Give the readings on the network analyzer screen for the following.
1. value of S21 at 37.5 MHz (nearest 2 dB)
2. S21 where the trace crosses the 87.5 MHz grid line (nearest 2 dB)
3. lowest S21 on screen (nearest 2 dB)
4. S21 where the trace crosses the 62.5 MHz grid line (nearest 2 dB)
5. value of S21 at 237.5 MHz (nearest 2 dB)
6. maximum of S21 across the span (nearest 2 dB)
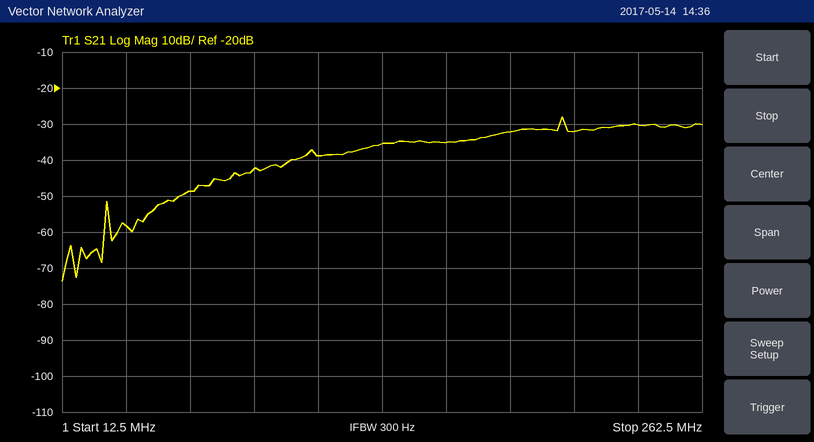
-58 dB
-42 dB
-74 dB
-48 dB
-30 dB
-28 dB
